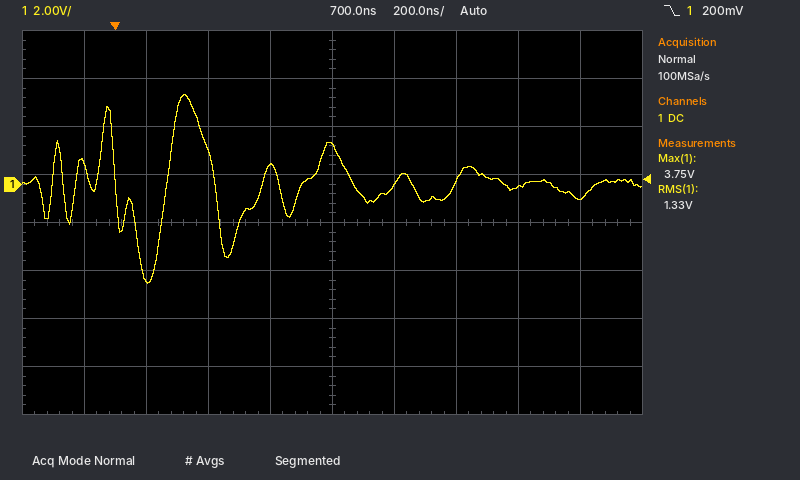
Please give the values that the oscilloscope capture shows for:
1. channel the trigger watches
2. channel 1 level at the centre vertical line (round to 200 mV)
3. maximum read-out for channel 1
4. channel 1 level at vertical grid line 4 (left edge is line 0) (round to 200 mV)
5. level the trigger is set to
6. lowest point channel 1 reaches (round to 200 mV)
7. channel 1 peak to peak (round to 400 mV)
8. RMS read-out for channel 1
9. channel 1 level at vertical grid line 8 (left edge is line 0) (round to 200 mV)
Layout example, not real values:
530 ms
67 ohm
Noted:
channel 1
1.6 V
3.75 V
800 mV
200 mV
-4.2 V
8.0 V
1.33 V
-200 mV
